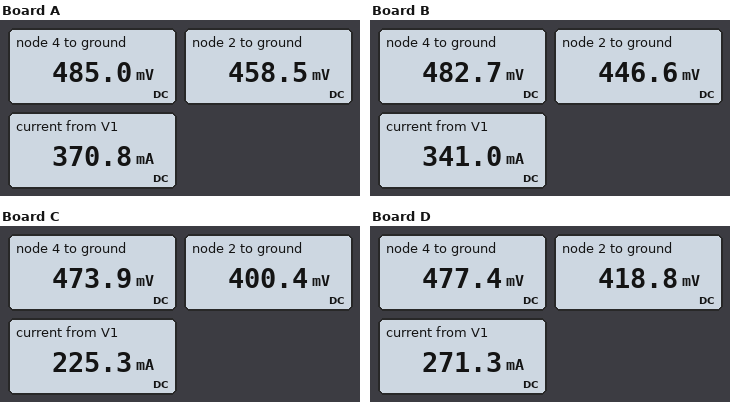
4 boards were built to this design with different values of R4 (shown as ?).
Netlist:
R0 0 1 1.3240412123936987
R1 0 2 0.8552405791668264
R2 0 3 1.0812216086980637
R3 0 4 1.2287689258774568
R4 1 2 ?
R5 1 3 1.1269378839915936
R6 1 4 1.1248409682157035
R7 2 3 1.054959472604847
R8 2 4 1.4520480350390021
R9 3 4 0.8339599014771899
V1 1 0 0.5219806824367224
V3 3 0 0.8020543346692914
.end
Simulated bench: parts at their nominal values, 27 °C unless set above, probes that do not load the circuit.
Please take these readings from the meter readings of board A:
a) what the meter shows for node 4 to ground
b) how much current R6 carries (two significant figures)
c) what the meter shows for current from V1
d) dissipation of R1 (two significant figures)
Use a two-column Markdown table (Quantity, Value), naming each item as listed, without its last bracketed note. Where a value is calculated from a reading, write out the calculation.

| Quantity | Value |
|---|---|
| what the meter shows for node 4 to ground | 485.0 mV |
| how much current R6 carries | (522 mV - 485 mV) / 1.125 Ω = 33 mA |
| what the meter shows for current from V1 | 370.8 mA |
| dissipation of R1 | (458.5 mV)^2 / 855.2 mΩ = 250 mW |
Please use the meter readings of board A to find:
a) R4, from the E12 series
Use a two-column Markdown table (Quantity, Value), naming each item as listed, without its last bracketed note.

| Quantity | Value |
|---|---|
| R4, from the E12 series | 0.33 Ω |
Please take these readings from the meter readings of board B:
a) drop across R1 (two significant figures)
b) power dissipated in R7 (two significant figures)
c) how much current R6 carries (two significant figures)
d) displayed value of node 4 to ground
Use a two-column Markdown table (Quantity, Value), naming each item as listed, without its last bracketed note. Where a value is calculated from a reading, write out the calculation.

| Quantity | Value |
|---|---|
| drop across R1 | 446.6 mV = 450 mV |
| power dissipated in R7 | (802.1 mV - 446.6 mV)^2 / 1.055 Ω = 120 mW |
| how much current R6 carries | (522 mV - 482.7 mV) / 1.125 Ω = 35 mA |
| displayed value of node 4 to ground | 482.7 mV |
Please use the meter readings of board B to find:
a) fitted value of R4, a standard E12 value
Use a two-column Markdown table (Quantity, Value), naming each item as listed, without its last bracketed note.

| Quantity | Value |
|---|---|
| fitted value of R4, a standard E12 value | 0.47 Ω |
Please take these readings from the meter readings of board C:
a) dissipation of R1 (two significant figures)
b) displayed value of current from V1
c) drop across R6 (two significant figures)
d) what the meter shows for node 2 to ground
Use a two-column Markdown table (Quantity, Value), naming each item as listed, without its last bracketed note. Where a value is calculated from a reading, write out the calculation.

| Quantity | Value |
|---|---|
| dissipation of R1 | (400.4 mV)^2 / 855.2 mΩ = 190 mW |
| displayed value of current from V1 | 225.3 mA |
| drop across R6 | 522 mV - 473.9 mV = 48 mV |
| what the meter shows for node 2 to ground | 400.4 mV |
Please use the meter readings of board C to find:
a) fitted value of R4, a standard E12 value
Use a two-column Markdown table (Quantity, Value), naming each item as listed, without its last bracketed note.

| Quantity | Value |
|---|---|
| fitted value of R4, a standard E12 value | 3.3 Ω |
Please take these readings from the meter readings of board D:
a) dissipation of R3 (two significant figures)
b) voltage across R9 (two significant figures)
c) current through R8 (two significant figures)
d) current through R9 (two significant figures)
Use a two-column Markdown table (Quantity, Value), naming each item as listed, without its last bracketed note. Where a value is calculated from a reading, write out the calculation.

| Quantity | Value |
|---|---|
| dissipation of R3 | (477.4 mV)^2 / 1.229 Ω = 190 mW |
| voltage across R9 | 802.1 mV - 477.4 mV = 320 mV |
| current through R8 | (477.4 mV - 418.8 mV) / 1.452 Ω = 40 mA |
| current through R9 | (802.1 mV - 477.4 mV) / 834 mΩ = 390 mA |
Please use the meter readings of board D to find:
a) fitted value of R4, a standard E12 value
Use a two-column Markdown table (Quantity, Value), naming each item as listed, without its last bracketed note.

| Quantity | Value |
|---|---|
| fitted value of R4, a standard E12 value | 1.2 Ω |
